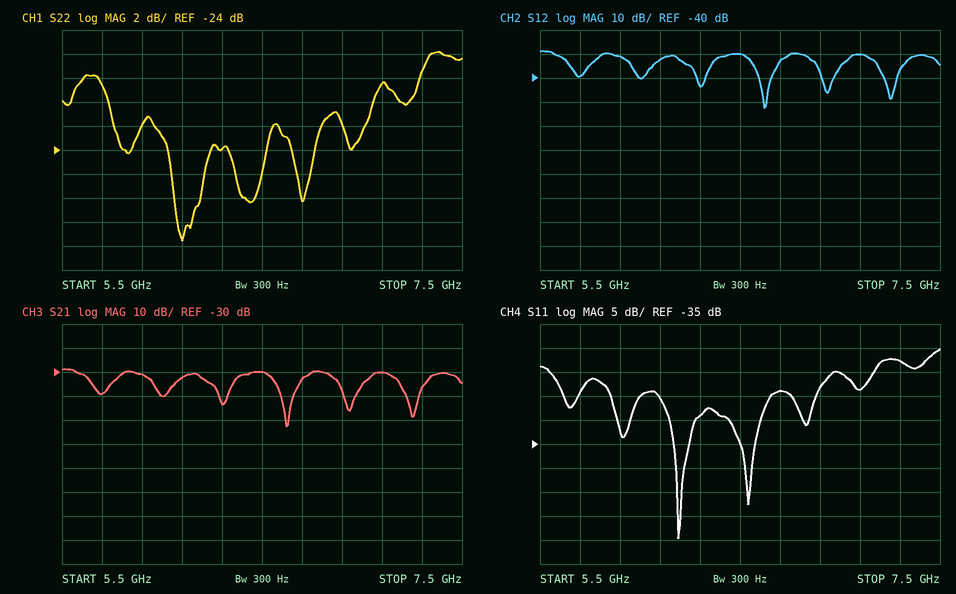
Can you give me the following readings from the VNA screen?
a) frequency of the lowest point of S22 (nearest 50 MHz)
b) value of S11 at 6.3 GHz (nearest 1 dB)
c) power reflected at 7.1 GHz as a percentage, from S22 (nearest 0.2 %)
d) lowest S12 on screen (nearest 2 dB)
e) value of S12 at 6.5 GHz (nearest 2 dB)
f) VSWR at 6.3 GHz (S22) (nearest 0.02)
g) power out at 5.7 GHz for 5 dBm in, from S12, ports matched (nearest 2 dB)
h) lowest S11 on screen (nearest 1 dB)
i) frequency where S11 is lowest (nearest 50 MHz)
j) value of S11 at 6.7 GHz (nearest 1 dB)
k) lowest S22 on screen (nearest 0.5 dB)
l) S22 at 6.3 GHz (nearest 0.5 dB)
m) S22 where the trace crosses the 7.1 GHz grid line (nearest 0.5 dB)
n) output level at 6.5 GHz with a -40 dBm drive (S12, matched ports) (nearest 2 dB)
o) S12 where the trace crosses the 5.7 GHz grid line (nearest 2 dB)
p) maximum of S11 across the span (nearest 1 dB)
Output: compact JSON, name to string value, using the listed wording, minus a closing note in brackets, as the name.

{"frequency of the lowest point of S22": "6.10 GHz", "value of S11 at 6.3 GHz": "-29 dB", "power reflected at 7.1 GHz as a percentage, from S22": "1.4 %", "lowest S12 on screen": "-52 dB", "value of S12 at 6.5 GHz": "-30 dB", "VSWR at 6.3 GHz (S22)": "1.14", "power out at 5.7 GHz for 5 dBm in, from S12, ports matched": "-34 dBm", "lowest S11 on screen": "-55 dB", "frequency where S11 is lowest": "6.20 GHz", "value of S11 at 6.7 GHz": "-24 dB", "lowest S22 on screen": "-31.5 dB", "S22 at 6.3 GHz": "-24.0 dB", "S22 where the trace crosses the 7.1 GHz grid line": "-18.5 dB", "output level at 6.5 GHz with a -40 dBm drive (S12, matched ports)": "-70 dBm", "S12 where the trace crosses the 5.7 GHz grid line": "-40 dB", "maximum of S11 across the span": "-15 dB"}
